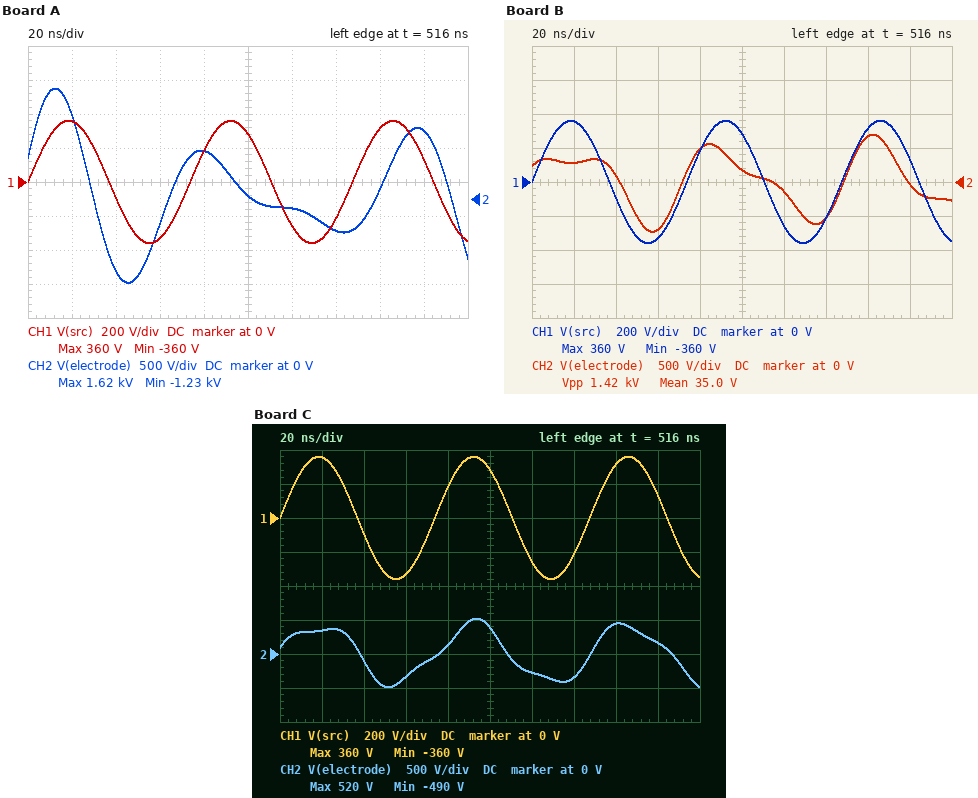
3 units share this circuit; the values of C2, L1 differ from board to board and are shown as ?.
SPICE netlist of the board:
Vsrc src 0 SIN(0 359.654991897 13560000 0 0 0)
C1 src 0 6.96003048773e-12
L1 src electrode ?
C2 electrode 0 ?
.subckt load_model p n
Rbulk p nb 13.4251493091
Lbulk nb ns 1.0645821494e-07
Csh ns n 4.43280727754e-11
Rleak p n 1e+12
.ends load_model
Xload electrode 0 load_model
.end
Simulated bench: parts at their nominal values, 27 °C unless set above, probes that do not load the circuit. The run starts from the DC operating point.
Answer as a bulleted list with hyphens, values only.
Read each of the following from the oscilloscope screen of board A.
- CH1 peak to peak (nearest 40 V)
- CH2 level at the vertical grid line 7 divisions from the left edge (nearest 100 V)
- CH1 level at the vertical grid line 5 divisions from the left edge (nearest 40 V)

- 720 V
- -500 V
- 280 V
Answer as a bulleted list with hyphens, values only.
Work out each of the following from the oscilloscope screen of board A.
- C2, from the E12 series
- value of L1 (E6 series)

- 2.7 nF
- 33 nH
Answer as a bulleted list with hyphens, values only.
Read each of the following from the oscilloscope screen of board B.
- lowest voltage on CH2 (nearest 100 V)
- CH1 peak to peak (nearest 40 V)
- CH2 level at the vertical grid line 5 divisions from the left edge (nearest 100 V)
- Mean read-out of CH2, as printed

- -700 V
- 720 V
- 200 V
- 35.0 V
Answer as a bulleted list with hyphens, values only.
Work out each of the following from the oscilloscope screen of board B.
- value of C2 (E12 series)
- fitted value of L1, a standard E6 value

- 1.2 nF
- 33 nH
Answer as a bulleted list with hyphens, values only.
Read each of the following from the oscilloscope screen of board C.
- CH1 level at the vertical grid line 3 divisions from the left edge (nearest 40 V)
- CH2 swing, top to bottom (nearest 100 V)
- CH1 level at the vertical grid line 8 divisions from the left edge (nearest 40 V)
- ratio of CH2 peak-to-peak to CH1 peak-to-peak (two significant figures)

- -320 V
- 1.0 kV
- 320 V
- 1.4
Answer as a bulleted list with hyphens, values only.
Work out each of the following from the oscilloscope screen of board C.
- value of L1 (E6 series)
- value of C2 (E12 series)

- 33 nH
- 680 pF
